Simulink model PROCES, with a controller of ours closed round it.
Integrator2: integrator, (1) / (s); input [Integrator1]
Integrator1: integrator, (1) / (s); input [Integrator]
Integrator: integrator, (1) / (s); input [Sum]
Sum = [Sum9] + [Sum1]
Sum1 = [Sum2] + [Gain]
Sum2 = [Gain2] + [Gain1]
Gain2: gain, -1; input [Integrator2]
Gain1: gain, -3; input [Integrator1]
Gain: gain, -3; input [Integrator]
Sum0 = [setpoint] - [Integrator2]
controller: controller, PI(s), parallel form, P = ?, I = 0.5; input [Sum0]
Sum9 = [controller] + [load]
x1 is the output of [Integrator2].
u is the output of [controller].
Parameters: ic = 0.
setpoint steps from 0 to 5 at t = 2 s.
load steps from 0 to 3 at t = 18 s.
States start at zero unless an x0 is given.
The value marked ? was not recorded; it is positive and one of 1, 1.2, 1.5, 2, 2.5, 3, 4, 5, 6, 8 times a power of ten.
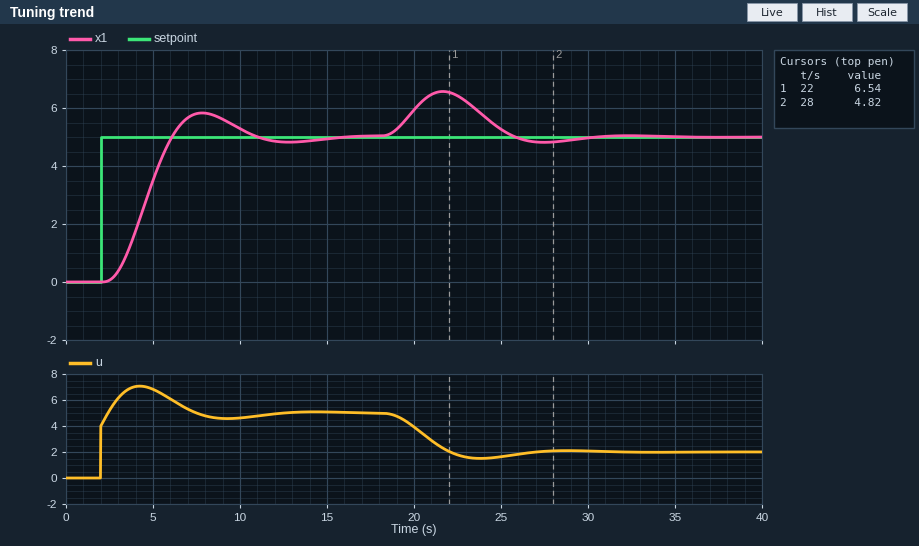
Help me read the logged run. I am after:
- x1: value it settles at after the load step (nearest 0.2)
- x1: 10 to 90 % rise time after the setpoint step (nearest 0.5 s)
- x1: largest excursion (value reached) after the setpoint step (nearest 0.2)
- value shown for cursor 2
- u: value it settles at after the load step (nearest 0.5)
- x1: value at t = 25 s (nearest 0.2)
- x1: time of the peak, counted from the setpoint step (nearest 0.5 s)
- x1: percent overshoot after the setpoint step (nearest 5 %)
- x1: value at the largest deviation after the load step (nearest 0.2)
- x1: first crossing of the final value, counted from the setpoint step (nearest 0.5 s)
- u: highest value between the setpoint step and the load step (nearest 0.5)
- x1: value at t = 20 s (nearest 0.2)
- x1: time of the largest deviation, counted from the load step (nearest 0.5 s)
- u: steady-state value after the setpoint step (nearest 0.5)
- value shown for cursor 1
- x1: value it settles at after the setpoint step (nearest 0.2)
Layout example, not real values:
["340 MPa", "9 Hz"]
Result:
["5.0", "2.5 s", "5.8", "4.82", "2.0", "5.2", "6.0 s", "15 %", "6.6", "4.0 s", "7.0", "6.0", "3.5 s", "5.0", "6.54", "5.0"]
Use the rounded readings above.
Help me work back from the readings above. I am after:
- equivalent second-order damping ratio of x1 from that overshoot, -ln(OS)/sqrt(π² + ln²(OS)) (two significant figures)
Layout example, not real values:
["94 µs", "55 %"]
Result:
["0.52"]
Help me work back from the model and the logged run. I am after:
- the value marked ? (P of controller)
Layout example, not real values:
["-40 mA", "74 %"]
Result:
["0.8"]
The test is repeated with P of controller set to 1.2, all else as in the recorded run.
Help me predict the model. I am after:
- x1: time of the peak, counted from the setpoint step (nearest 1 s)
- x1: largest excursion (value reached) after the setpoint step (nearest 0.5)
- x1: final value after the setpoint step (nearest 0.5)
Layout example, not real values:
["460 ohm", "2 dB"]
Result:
["5 s", "5.5", "5.0"]
